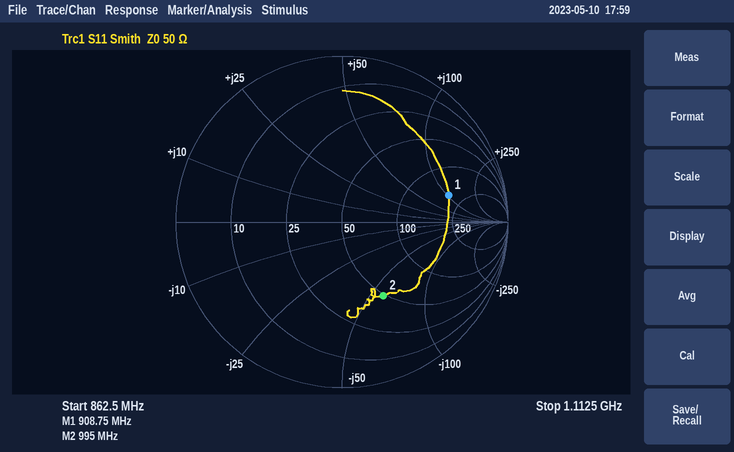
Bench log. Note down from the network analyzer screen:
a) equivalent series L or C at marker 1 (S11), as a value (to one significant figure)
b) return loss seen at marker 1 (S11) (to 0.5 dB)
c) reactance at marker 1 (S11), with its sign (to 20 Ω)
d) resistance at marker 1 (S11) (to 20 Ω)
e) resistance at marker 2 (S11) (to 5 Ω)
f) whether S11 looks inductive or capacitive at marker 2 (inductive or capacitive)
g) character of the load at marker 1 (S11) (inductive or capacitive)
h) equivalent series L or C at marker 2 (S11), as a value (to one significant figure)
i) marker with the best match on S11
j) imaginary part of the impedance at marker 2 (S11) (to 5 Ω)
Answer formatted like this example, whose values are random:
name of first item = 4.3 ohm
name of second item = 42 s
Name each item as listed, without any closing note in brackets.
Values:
equivalent series L or C at marker 1 (S11), as a value = 20 nH
return loss seen at marker 1 (S11) = 3.5 dB
reactance at marker 1 (S11), with its sign = +100 Ω
resistance at marker 1 (S11) = 180 Ω
resistance at marker 2 (S11) = 50 Ω
whether S11 looks inductive or capacitive at marker 2 = capacitive
character of the load at marker 1 (S11) = inductive
equivalent series L or C at marker 2 (S11), as a value = 3 pF
marker with the best match on S11 = marker 2
imaginary part of the impedance at marker 2 (S11) = -60 Ω
